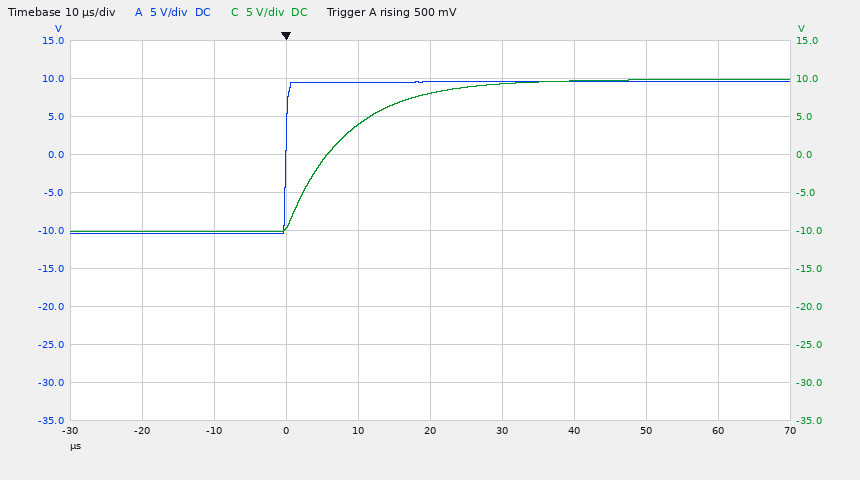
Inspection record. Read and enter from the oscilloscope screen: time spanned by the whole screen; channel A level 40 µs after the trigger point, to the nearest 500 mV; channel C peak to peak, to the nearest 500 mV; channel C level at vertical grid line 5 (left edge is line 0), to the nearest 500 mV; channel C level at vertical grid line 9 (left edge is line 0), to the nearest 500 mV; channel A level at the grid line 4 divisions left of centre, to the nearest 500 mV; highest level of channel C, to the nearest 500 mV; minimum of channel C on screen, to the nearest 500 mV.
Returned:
100 µs
9.5 V
20.0 V
8.0 V
10.0 V
-10.5 V
10.0 V
-10.0 V
